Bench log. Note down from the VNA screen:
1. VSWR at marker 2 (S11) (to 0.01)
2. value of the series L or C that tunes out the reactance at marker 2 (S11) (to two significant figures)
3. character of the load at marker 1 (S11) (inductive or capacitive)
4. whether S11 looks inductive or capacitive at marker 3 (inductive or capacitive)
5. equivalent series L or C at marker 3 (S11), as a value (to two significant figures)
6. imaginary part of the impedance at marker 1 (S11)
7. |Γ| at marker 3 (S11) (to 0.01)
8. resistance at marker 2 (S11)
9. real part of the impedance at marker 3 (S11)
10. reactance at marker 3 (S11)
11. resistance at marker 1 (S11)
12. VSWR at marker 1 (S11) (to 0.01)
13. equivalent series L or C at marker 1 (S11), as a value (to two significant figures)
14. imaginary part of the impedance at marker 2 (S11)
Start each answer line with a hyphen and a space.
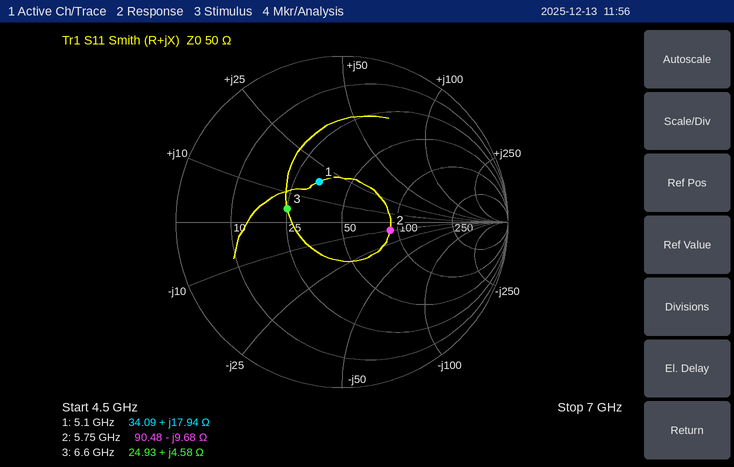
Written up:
- 1.84
- 270 pH
- inductive
- inductive
- 110 pH
- +17.94 Ω
- 0.34
- 90.48 Ω
- 24.93 Ω
- +4.58 Ω
- 34.09 Ω
- 1.77
- 560 pH
- -9.68 Ω
